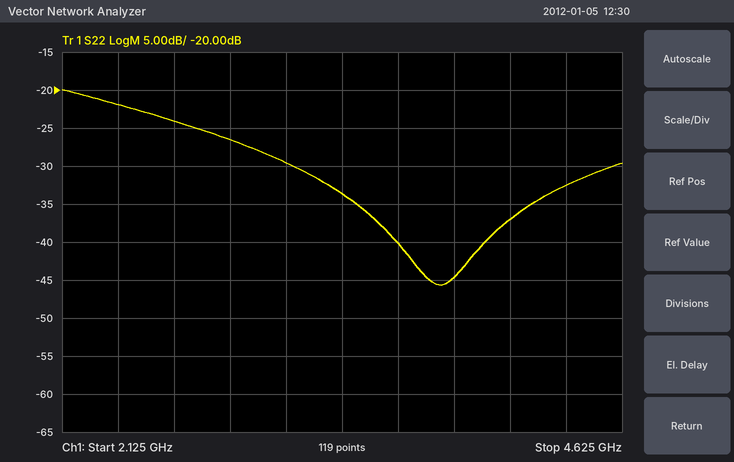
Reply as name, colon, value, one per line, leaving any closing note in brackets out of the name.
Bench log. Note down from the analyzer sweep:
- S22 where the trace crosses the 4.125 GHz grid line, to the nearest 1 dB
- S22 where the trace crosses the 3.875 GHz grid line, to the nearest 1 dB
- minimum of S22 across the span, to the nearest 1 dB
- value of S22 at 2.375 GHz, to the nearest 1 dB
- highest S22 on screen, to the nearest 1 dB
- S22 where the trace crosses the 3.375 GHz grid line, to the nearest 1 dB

S22 where the trace crosses the 4.125 GHz grid line, to the nearest 1 dB: -37 dB
S22 where the trace crosses the 3.875 GHz grid line, to the nearest 1 dB: -45 dB
minimum of S22 across the span, to the nearest 1 dB: -46 dB
value of S22 at 2.375 GHz, to the nearest 1 dB: -22 dB
highest S22 on screen, to the nearest 1 dB: -20 dB
S22 where the trace crosses the 3.375 GHz grid line, to the nearest 1 dB: -34 dB
